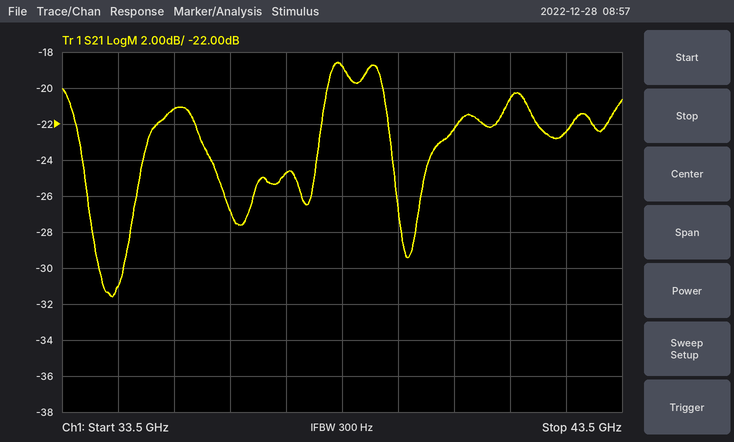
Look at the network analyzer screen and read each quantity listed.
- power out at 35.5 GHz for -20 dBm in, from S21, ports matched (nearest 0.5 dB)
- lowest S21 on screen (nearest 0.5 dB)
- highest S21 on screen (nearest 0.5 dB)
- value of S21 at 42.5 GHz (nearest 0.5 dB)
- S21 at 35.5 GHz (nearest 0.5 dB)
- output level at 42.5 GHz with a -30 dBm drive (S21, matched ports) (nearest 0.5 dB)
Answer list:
-41.0 dBm
-31.5 dB
-18.5 dB
-22.5 dB
-21.0 dB
-52.5 dBm
